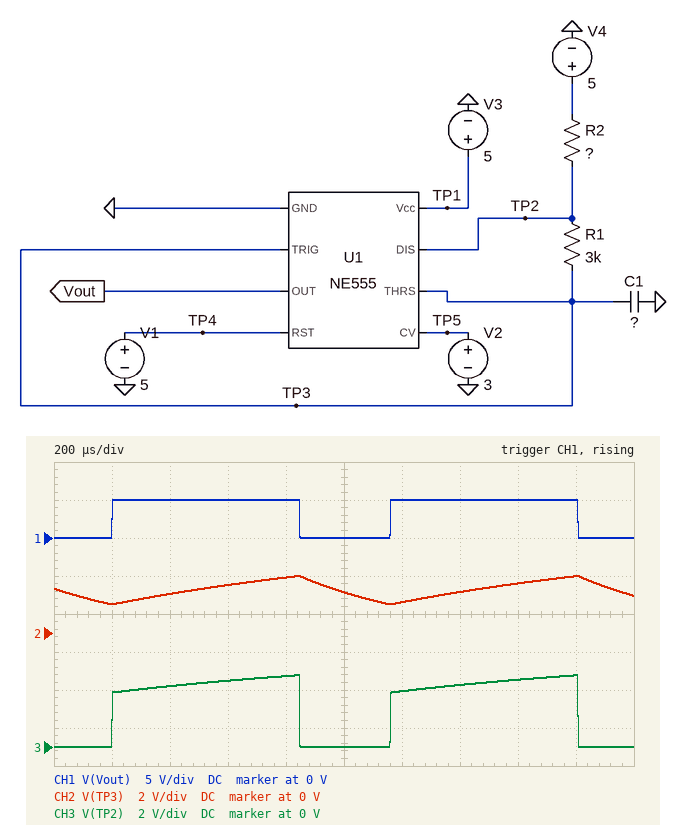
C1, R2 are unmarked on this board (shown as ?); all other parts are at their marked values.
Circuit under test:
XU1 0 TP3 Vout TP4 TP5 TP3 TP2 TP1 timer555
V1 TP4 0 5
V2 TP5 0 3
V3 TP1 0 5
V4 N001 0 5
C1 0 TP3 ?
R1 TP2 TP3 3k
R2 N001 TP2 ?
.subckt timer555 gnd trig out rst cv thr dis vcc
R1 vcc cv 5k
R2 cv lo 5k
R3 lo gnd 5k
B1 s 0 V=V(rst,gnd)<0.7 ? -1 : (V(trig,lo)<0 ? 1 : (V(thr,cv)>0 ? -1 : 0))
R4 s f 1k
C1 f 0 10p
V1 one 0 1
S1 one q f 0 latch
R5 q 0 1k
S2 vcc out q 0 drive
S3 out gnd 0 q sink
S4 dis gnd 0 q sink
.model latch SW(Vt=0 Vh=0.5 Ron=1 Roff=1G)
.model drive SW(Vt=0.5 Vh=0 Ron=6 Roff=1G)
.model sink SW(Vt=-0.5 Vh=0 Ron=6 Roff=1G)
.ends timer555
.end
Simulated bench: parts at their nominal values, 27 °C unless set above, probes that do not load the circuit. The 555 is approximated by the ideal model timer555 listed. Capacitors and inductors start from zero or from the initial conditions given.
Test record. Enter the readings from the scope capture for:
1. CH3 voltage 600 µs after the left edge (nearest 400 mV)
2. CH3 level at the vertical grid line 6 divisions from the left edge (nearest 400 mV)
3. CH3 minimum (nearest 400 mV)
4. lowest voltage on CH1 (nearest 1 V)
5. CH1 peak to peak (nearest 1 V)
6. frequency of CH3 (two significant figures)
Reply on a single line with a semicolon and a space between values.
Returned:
3.6 V; 2.8 V; 0 V; 0 V; 5 V; 1.0 kHz
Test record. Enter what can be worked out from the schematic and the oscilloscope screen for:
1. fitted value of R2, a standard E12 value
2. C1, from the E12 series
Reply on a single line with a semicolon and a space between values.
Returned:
4.7 kΩ; 150 nF
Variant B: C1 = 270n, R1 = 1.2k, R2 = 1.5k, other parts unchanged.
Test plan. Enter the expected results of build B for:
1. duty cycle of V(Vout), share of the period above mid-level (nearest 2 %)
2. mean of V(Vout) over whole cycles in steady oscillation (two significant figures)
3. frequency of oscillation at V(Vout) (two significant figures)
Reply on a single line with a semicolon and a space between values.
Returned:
64 %; 3.2 V; 1.6 kHz
